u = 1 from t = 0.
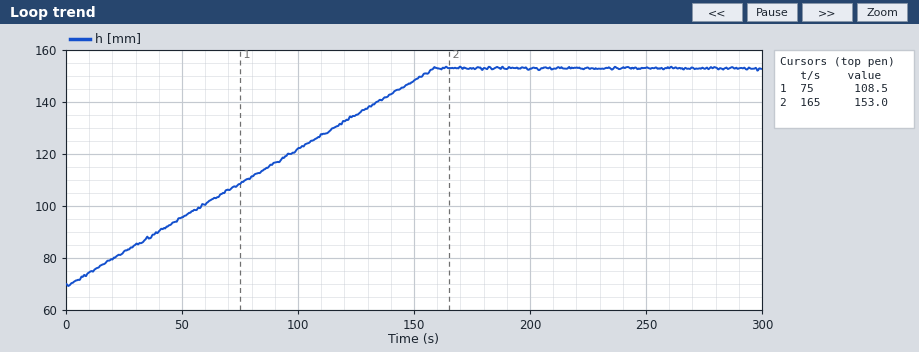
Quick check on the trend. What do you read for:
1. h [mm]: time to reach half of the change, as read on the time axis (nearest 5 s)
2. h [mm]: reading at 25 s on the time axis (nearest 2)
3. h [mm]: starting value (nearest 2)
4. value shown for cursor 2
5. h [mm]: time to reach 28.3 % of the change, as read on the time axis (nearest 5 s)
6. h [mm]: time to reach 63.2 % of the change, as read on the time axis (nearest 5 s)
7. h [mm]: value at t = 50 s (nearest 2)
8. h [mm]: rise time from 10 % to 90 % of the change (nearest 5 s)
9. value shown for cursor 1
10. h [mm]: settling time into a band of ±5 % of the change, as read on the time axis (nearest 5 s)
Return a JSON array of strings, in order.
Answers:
["80 s", "82", "70", "153.0", "45 s", "100 s", "96", "125 s", "108.5", "150 s"]
